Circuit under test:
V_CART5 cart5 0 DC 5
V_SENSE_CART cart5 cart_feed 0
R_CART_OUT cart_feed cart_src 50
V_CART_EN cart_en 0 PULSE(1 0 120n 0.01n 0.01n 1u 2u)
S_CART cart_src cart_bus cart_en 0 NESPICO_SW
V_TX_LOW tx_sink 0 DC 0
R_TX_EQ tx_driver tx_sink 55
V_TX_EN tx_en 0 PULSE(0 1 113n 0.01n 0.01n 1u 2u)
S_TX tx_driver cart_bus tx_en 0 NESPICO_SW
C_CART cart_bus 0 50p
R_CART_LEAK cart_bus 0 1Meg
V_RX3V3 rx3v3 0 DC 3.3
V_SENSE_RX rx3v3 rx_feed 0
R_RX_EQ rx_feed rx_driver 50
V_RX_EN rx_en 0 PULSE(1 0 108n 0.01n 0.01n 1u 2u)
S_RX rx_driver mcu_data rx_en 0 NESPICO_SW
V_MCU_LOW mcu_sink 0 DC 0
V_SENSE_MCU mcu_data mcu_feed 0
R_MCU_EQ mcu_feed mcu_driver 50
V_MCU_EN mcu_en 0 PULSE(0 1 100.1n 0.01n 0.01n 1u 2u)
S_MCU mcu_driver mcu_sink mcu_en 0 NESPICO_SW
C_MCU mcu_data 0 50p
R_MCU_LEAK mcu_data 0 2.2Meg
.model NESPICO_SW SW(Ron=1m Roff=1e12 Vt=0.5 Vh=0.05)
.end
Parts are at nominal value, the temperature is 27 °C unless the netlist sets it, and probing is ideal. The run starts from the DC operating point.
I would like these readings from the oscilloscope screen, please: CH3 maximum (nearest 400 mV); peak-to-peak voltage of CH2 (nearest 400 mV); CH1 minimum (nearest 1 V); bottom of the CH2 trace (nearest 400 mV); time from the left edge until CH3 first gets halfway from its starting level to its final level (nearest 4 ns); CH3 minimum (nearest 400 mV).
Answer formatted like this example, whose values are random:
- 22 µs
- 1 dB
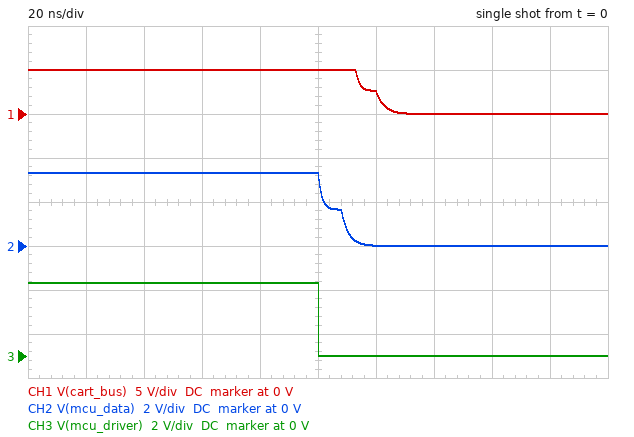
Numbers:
- 3.2 V
- 3.2 V
- 0 V
- 0 V
- 100 ns
- 0 V
